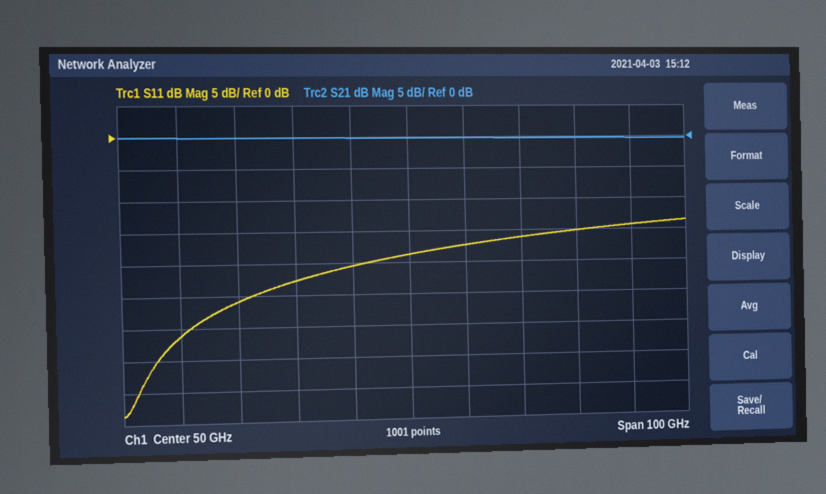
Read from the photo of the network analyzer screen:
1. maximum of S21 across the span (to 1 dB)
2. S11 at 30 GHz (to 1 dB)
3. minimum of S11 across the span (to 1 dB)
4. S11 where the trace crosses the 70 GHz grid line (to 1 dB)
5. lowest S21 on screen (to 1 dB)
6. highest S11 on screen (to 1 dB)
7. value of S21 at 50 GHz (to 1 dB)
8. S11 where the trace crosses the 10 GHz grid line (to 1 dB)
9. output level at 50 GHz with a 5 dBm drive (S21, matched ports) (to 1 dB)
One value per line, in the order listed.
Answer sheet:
0 dB
-23 dB
-44 dB
-16 dB
0 dB
-14 dB
0 dB
-31 dB
5 dBm
